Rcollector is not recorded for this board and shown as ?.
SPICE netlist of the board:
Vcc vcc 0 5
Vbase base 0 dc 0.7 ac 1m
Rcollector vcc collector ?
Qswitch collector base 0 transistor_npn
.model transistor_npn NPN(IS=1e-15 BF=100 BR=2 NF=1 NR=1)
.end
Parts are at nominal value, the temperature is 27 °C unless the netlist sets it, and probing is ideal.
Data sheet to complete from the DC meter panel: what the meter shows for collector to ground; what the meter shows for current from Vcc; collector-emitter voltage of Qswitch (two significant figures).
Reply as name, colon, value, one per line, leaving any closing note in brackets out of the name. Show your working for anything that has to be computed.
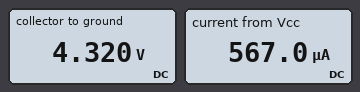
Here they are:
what the meter shows for collector to ground: 4.320 V
what the meter shows for current from Vcc: 567.0 µA
collector-emitter voltage of Qswitch: 4.32 V = 4.3 V
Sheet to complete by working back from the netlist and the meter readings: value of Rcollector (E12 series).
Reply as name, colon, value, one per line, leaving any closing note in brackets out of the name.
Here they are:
value of Rcollector: 1.2 kΩ
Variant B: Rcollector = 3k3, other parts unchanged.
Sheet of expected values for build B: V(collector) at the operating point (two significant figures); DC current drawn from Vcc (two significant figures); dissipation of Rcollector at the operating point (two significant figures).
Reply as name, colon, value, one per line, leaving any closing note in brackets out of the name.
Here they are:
V(collector) at the operating point: 3.1 V
DC current drawn from Vcc: 570 µA
dissipation of Rcollector at the operating point: 1.1 mW
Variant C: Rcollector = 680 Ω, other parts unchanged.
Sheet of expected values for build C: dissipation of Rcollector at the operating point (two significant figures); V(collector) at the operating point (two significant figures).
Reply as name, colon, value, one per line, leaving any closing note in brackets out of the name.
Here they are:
dissipation of Rcollector at the operating point: 220 µW
V(collector) at the operating point: 4.6 V
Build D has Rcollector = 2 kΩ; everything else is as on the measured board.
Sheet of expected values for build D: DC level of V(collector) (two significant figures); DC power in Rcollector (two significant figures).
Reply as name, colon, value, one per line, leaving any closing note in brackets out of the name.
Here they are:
DC level of V(collector): 3.9 V
DC power in Rcollector: 640 µW
